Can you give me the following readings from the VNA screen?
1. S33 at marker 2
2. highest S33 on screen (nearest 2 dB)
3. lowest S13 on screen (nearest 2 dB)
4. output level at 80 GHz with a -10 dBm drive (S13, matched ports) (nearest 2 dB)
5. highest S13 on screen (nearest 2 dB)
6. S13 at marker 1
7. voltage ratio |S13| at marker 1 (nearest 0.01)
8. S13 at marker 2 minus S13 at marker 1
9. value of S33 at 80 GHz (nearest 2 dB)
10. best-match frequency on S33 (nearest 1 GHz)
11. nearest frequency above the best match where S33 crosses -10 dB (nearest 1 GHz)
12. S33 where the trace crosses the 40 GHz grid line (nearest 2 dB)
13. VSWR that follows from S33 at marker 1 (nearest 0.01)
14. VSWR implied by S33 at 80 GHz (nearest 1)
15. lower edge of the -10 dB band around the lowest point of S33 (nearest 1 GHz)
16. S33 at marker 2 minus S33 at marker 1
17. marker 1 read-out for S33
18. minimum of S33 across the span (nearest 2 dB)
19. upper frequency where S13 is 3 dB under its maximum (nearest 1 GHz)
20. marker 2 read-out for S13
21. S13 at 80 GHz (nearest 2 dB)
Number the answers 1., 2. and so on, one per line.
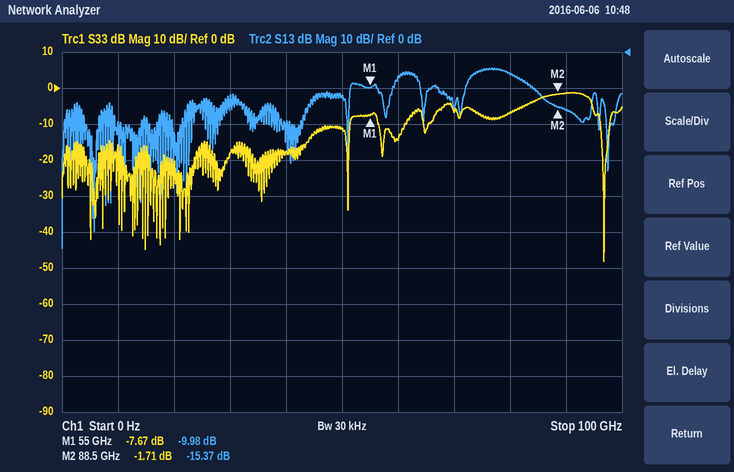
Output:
1. -1.71 dB
2. -2 dB
3. -54 dB
4. -16 dBm
5. -4 dB
6. -9.98 dB
7. 0.32
8. -5.39 dB
9. -6 dB
10. 97 GHz
11. 98 GHz
12. -18 dB
13. 2.41
14. 3
15. 96 GHz
16. 5.96 dB
17. -7.67 dB
18. -48 dB
19. 82 GHz
20. -15.37 dB
21. -6 dB
